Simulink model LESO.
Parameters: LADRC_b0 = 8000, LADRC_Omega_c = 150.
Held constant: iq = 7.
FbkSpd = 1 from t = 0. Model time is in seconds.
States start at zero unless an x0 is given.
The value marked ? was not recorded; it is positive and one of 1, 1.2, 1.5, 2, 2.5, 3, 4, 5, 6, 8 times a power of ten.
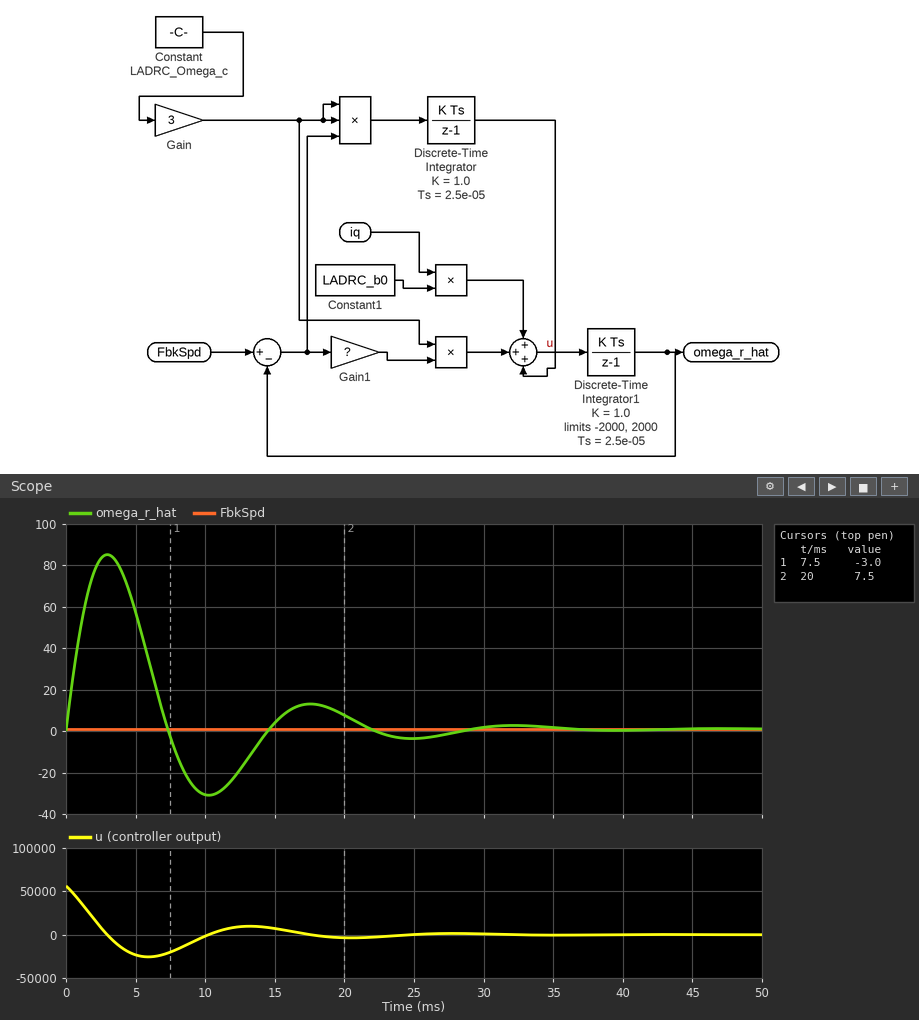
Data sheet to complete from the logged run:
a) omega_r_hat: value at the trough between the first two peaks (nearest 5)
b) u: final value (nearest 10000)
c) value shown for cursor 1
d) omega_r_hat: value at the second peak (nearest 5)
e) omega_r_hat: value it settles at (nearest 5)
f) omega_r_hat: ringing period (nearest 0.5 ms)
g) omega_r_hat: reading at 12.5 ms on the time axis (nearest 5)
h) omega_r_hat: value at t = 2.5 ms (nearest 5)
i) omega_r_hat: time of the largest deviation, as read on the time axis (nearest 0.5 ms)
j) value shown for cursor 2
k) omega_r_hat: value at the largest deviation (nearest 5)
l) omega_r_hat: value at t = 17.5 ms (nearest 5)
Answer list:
-30
0
-3.0
15
0
14.5 ms
-20
85
3.0 ms
7.5
85
15
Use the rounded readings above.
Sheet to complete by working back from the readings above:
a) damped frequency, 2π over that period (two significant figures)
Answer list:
0.43 rad/ms
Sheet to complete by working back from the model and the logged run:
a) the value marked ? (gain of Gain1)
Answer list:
0.6
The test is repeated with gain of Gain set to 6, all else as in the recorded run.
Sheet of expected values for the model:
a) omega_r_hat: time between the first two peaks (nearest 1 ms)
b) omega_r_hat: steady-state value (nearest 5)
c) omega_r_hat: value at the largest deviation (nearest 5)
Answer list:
7 ms
0
45
